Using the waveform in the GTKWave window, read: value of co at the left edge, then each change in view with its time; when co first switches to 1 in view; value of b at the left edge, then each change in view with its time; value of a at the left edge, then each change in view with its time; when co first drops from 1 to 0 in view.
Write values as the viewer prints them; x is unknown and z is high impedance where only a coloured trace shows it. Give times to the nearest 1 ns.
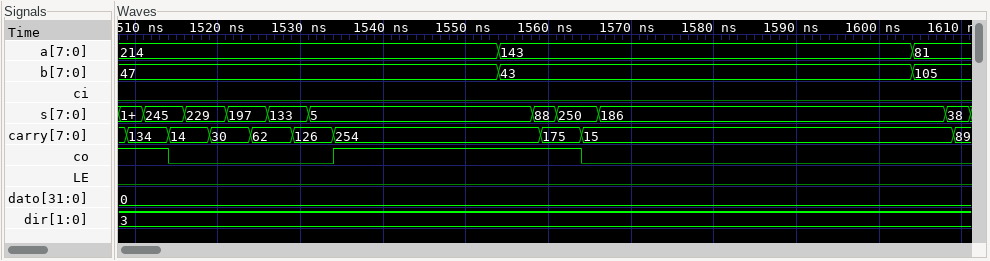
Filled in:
1, 0 at 1514 ns, 1 at 1534 ns, 0 at 1564 ns
1534 ns
47, 43 at 1554 ns, 105 at 1604 ns
214, 143 at 1554 ns, 81 at 1604 ns
1514 ns
